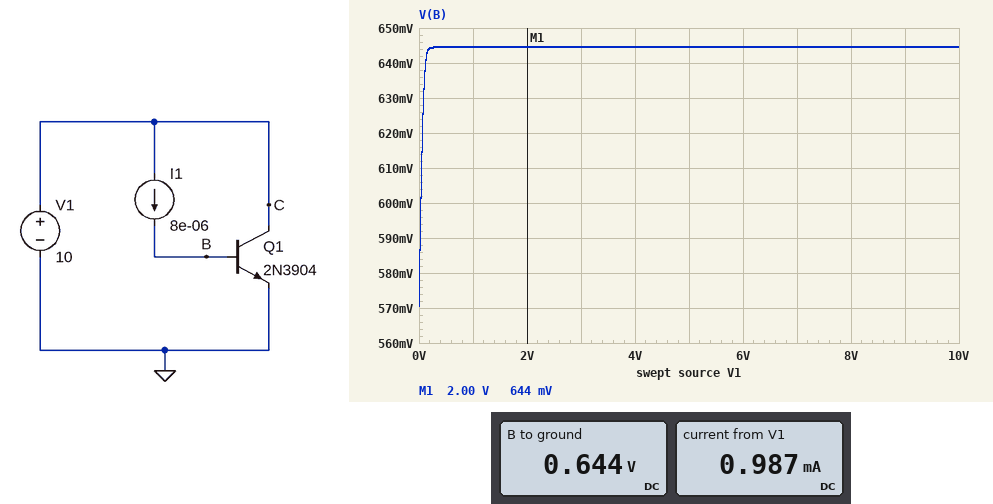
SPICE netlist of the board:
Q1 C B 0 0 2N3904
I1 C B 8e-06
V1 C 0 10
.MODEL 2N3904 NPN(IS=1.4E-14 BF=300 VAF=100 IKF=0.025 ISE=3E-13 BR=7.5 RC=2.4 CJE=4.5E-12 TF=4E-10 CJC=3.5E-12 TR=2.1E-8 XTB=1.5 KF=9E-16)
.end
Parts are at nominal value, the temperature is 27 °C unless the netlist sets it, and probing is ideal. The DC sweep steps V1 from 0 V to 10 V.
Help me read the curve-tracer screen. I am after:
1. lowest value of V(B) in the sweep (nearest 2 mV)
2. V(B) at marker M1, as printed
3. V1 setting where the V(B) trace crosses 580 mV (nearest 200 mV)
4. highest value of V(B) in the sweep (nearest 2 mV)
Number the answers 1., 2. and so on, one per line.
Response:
1. 570 mV
2. 644 mV
3. 0 V
4. 644 mV
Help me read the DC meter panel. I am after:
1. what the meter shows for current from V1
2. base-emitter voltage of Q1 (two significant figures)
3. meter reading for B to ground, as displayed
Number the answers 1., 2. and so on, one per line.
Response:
1. 0.987 mA
2. 640 mV
3. 0.644 V
